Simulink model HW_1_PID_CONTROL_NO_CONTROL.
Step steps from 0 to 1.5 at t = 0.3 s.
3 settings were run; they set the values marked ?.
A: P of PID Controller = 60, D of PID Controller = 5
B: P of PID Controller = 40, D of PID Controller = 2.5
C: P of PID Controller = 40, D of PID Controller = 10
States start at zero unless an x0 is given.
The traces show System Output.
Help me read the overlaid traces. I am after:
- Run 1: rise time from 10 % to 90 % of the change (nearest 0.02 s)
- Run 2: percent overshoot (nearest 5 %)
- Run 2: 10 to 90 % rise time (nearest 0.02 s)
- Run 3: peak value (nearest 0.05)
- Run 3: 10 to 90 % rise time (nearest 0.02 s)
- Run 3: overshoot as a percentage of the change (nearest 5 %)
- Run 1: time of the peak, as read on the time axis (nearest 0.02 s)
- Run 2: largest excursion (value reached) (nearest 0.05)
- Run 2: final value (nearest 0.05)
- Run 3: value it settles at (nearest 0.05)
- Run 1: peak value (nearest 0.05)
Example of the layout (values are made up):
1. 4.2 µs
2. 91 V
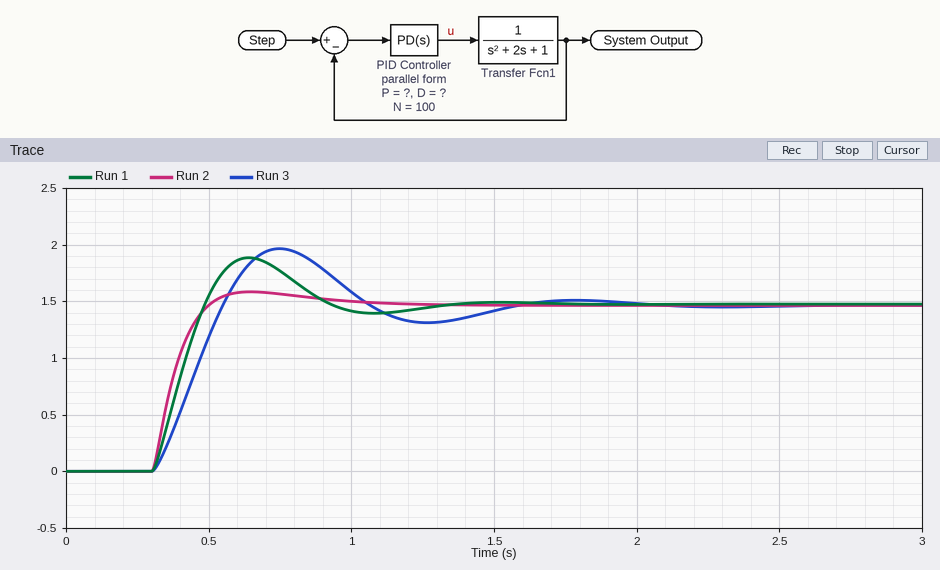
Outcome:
1. 0.14 s
2. 10 %
3. 0.14 s
4. 1.95
5. 0.18 s
6. 35 %
7. 0.64 s
8. 1.60
9. 1.45
10. 1.45
11. 1.90
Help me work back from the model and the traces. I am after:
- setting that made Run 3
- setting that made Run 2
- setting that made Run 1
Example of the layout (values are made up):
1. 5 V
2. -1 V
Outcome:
1. B
2. C
3. A
